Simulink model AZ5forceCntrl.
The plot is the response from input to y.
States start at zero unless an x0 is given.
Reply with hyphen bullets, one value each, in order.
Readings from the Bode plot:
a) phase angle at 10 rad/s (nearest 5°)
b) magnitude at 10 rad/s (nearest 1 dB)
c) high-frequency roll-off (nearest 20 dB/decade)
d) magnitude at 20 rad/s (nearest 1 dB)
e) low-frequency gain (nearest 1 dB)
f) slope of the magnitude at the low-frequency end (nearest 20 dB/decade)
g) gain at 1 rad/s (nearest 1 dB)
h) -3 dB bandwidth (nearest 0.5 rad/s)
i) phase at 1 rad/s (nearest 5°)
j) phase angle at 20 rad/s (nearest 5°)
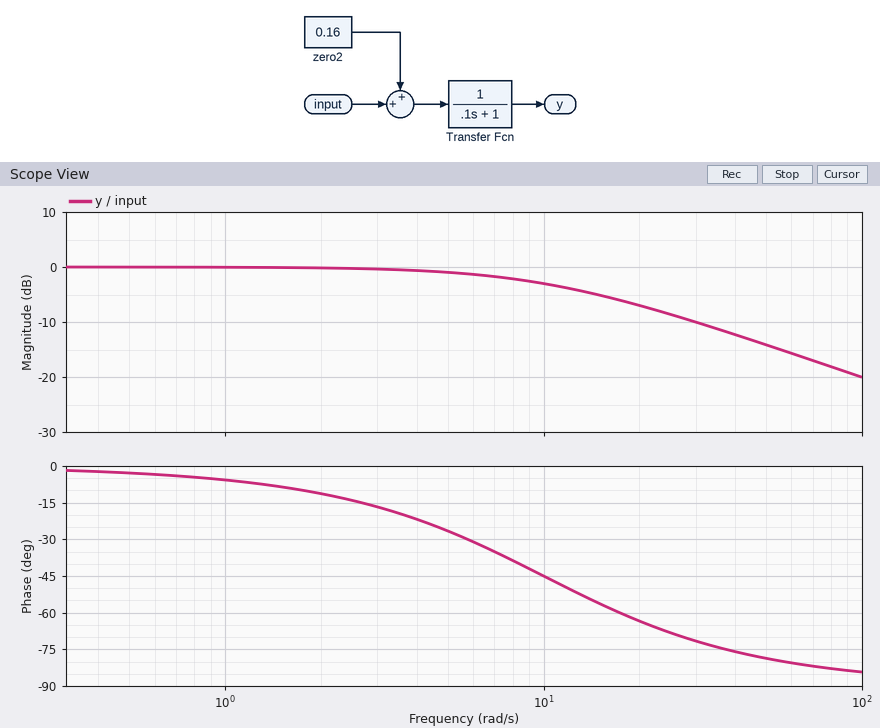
- -45°
- -3 dB
- -20 dB/decade
- -7 dB
- 0 dB
- 0 dB/decade
- 0 dB
- 10.0 rad/s
- -5°
- -65°
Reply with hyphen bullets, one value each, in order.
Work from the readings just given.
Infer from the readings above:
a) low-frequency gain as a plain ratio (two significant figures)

- 1.0
